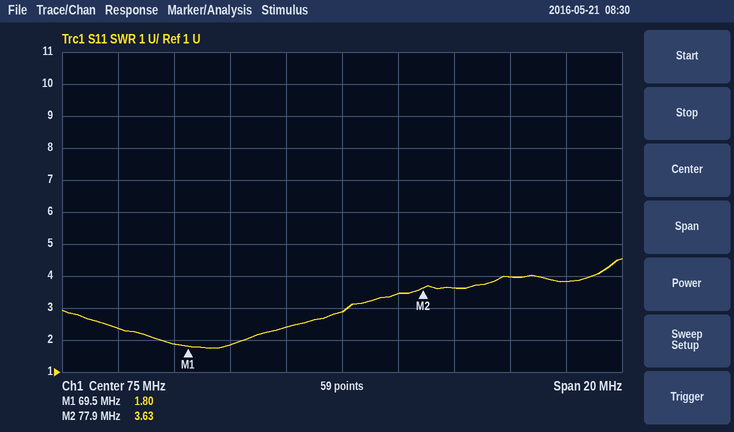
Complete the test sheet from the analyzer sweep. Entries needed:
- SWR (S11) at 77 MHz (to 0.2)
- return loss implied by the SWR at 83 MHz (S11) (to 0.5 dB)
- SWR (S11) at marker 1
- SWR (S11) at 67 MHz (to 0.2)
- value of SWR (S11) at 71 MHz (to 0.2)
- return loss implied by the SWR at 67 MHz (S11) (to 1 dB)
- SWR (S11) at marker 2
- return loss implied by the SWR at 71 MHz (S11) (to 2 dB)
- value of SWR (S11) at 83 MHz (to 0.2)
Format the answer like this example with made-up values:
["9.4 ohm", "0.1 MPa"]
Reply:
["3.4", "4.5 dB", "1.80", "2.4", "1.8", "8 dB", "3.63", "10 dB", "3.8"]
